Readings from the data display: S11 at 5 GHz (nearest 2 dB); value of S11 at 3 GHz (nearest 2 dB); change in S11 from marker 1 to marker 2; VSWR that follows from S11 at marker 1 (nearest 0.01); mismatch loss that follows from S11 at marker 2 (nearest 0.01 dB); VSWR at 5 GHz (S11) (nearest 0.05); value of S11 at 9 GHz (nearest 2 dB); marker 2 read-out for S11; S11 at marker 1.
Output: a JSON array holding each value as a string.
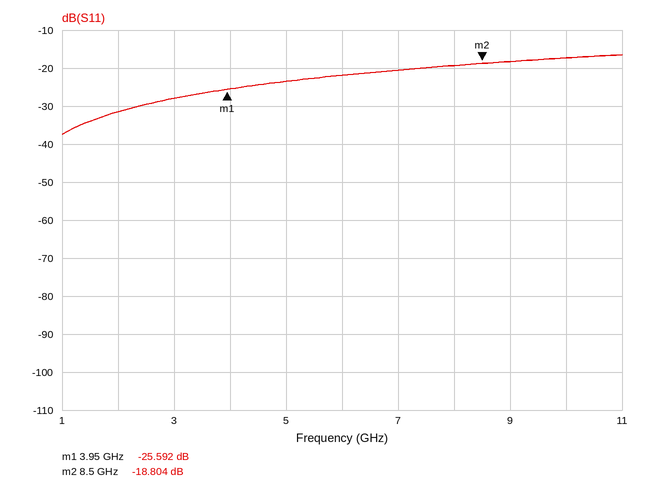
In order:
["-24 dB", "-28 dB", "6.788 dB", "1.11", "0.06 dB", "1.15", "-18 dB", "-18.804 dB", "-25.592 dB"]
